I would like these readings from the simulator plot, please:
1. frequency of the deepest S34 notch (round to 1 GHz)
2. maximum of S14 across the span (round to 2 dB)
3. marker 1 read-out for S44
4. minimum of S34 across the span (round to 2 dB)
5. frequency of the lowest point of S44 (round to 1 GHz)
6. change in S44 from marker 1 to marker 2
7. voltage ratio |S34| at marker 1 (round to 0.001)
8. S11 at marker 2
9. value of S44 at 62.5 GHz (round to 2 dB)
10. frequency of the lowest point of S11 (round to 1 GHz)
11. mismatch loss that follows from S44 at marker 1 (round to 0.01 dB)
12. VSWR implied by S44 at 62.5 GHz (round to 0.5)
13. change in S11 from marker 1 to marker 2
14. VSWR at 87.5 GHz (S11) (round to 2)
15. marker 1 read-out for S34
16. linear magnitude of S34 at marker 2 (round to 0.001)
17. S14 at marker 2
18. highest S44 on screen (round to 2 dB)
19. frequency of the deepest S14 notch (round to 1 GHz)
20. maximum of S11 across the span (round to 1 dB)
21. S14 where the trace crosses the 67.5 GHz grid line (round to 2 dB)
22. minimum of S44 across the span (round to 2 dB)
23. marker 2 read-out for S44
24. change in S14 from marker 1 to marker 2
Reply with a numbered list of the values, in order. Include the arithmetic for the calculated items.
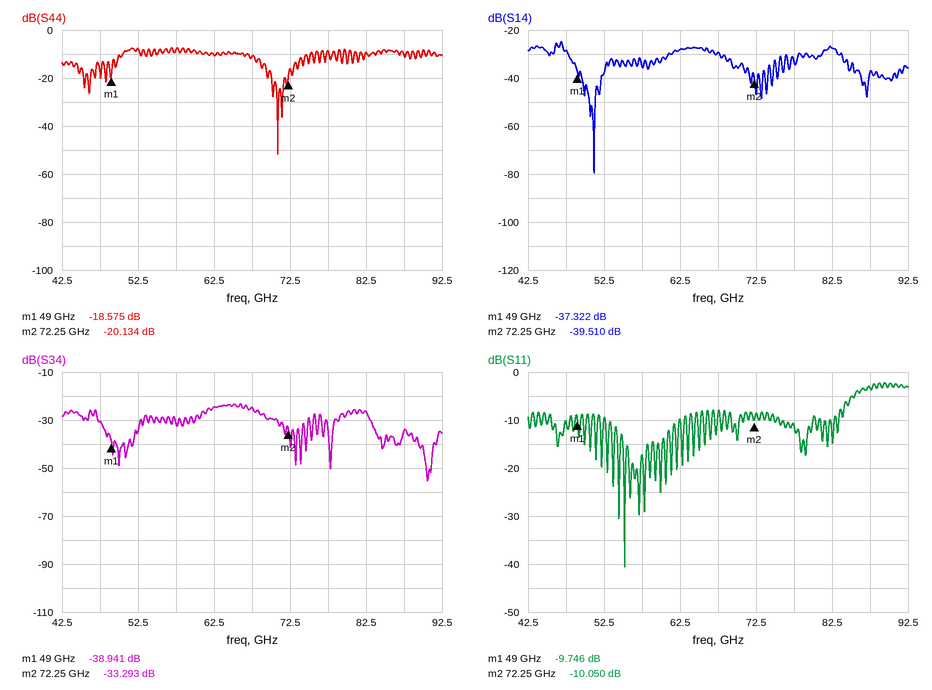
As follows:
1. 91 GHz
2. -24 dB
3. -18.575 dB
4. -56 dB
5. 71 GHz
6. -20.134 − (-18.575) = -1.559 dB
7. 10^(-38.941/20) ≈ 0.011
8. -10.050 dB
9. -10 dB
10. 55 GHz
11. −10 log10(1 − 10^(-18.575/10)) ≈ 0.06 dB
12. |Γ| = 10^(-10/20) = 0.3162; VSWR = (1 + 0.3162)/(1 − 0.3162) ≈ 1.92, so 2.0 to the nearest 0.5
13. -10.05 − (-9.746) = -0.304 dB
14. |Γ| = 10^(-3/20) = 0.7079; VSWR = (1 + 0.7079)/(1 − 0.7079) ≈ 6
15. -38.941 dB
16. 10^(-33.293/20) ≈ 0.022
17. -39.510 dB
18. -8 dB
19. 51 GHz
20. -2 dB
21. -30 dB
22. -52 dB
23. -20.134 dB
24. -39.51 − (-37.322) = -2.188 dB
